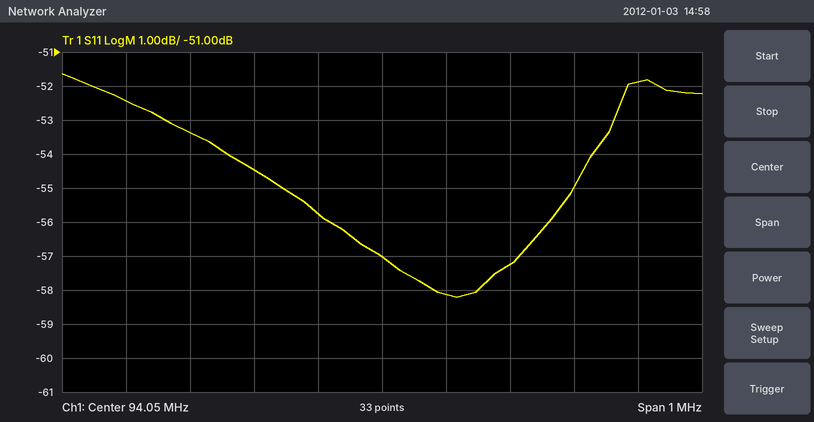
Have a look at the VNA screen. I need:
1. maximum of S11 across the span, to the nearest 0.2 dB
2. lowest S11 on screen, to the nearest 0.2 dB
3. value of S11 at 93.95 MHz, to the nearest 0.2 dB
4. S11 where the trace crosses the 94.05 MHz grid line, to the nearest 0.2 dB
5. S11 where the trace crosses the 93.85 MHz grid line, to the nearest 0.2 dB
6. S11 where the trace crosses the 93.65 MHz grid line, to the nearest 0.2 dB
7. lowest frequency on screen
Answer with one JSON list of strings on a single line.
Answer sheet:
["-51.6 dB", "-58.2 dB", "-55.8 dB", "-57.0 dB", "-54.4 dB", "-52.4 dB", "93.55 MHz"]
